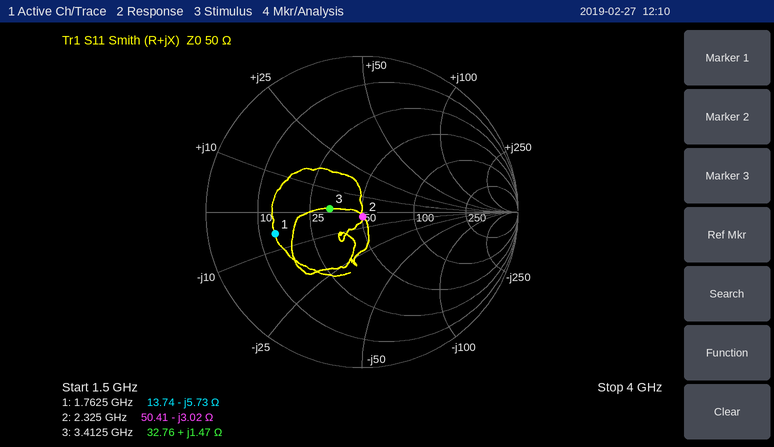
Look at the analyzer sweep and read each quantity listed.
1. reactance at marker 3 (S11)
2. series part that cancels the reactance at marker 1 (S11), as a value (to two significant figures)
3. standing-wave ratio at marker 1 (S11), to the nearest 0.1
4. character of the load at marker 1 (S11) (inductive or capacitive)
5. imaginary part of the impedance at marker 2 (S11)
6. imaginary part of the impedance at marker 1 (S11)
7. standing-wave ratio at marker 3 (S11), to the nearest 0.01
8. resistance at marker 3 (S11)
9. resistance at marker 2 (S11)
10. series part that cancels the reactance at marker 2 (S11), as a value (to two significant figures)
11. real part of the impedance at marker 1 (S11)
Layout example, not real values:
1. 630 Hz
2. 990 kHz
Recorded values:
1. +1.47 Ω
2. 520 pH
3. 3.7
4. capacitive
5. -3.02 Ω
6. -5.73 Ω
7. 1.53
8. 32.76 Ω
9. 50.41 Ω
10. 210 pH
11. 13.74 Ω
